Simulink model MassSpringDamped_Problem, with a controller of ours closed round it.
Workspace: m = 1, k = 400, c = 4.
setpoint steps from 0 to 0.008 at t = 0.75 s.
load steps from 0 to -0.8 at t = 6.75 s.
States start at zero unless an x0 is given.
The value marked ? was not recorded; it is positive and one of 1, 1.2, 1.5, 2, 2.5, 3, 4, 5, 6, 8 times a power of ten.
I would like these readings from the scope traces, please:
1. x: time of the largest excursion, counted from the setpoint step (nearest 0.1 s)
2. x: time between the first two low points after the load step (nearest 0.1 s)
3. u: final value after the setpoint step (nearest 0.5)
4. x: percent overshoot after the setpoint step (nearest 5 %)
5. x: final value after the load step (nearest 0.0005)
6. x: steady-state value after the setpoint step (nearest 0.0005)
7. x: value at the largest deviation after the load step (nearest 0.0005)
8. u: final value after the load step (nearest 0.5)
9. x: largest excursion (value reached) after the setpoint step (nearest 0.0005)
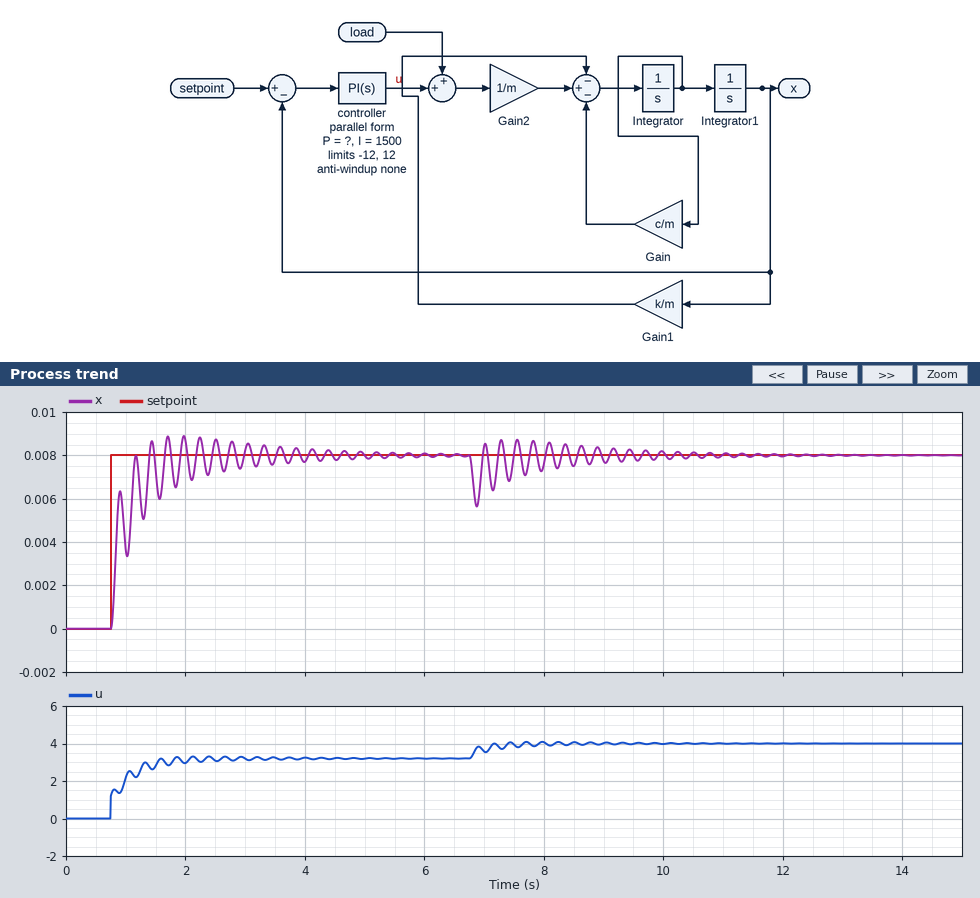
1.2 s
0.3 s
3.0
10 %
0.0080
0.0080
0.0055
4.0
0.0090
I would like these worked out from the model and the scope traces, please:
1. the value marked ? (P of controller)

150
